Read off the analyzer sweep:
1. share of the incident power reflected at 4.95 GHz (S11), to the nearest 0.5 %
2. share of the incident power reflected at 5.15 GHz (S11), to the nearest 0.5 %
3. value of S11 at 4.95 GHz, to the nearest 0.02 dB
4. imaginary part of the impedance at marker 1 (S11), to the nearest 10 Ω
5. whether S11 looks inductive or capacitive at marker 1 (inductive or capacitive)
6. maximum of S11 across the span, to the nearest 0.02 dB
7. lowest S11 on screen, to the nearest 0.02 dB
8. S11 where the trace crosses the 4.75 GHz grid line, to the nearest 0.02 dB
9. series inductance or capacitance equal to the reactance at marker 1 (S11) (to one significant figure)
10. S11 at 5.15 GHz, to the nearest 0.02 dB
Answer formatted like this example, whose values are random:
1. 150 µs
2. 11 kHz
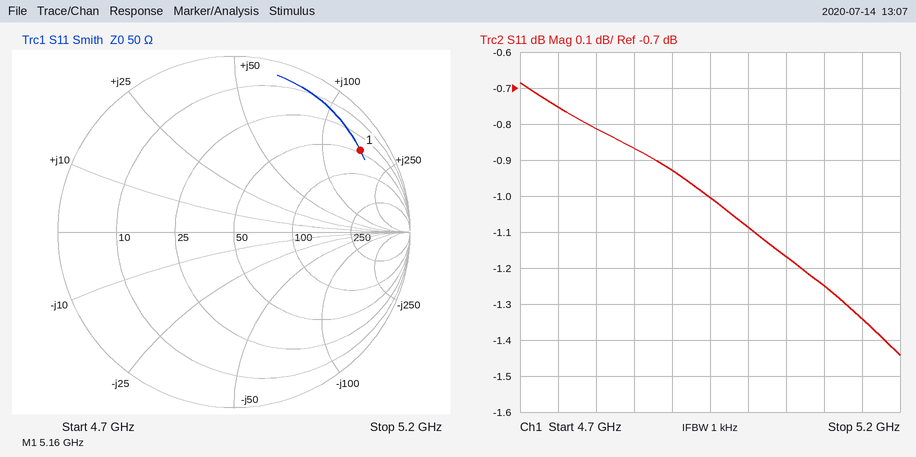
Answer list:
1. 79.5 %
2. 73.5 %
3. -1.00 dB
4. +160 Ω
5. inductive
6. -0.68 dB
7. -1.44 dB
8. -0.76 dB
9. 5 nH
10. -1.34 dB
